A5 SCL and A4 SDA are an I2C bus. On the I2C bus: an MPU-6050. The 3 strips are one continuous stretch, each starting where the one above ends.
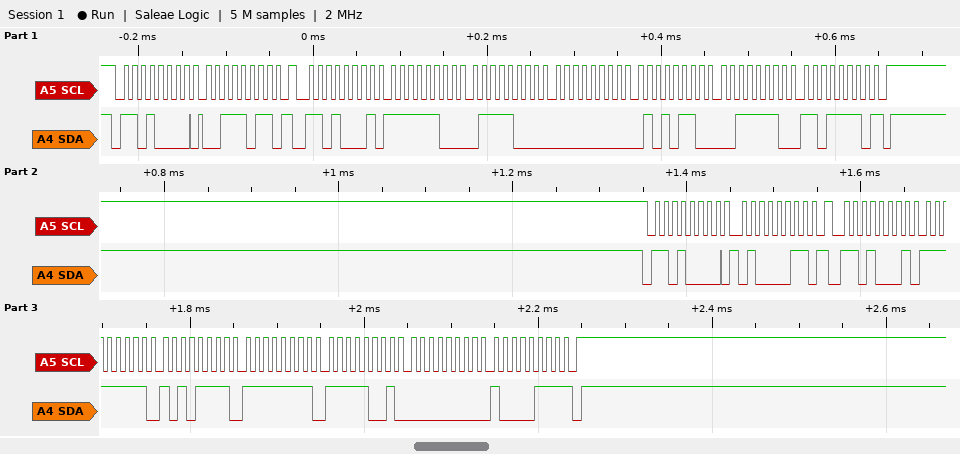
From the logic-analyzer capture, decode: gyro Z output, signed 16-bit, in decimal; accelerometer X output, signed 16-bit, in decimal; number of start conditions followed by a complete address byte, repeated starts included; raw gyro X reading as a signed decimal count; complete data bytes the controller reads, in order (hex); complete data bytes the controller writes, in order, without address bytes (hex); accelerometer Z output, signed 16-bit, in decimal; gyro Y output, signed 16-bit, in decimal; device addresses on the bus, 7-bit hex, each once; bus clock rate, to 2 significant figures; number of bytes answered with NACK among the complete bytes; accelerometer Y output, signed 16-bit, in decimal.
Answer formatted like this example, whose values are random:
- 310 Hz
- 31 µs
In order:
- 135
- -904
- 4
- -81
- FC 78 00 56 3E DE FF AF FF F9 00 87
- 3B 43
- 16094
- -7
- 0x68
- 100 kHz
- 2
- 86
